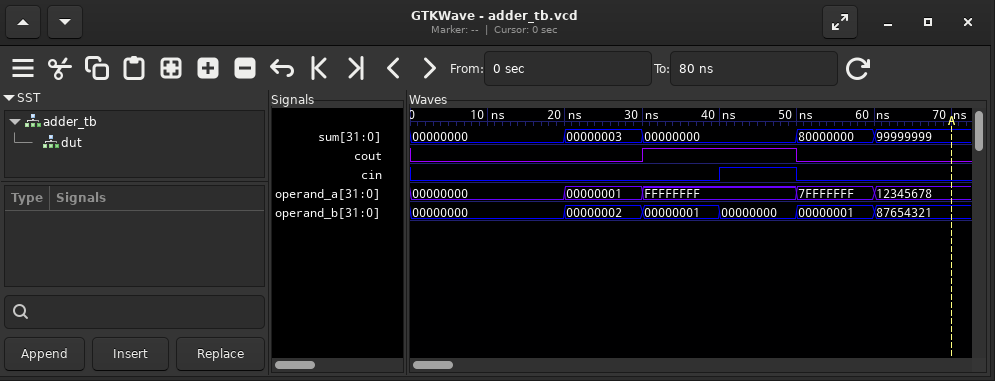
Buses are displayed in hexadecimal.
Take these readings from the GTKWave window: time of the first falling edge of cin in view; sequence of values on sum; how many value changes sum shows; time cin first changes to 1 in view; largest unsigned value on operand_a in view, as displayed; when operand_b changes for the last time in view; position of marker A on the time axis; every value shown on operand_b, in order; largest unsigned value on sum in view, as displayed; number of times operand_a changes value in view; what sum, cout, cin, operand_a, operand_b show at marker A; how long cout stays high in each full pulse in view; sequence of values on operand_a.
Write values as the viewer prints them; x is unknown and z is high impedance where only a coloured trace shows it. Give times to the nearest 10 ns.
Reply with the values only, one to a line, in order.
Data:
50 ns
00000000, 00000003, 00000000, 80000000, 99999999
4
40 ns
FFFFFFFF
60 ns
70 ns
00000000, 00000002, 00000001, 00000000, 00000001, 87654321
99999999
4
sum=99999999, cout=0, cin=0, operand_a=12345678, operand_b=87654321
20 ns
00000000, 00000001, FFFFFFFF, 7FFFFFFF, 12345678
